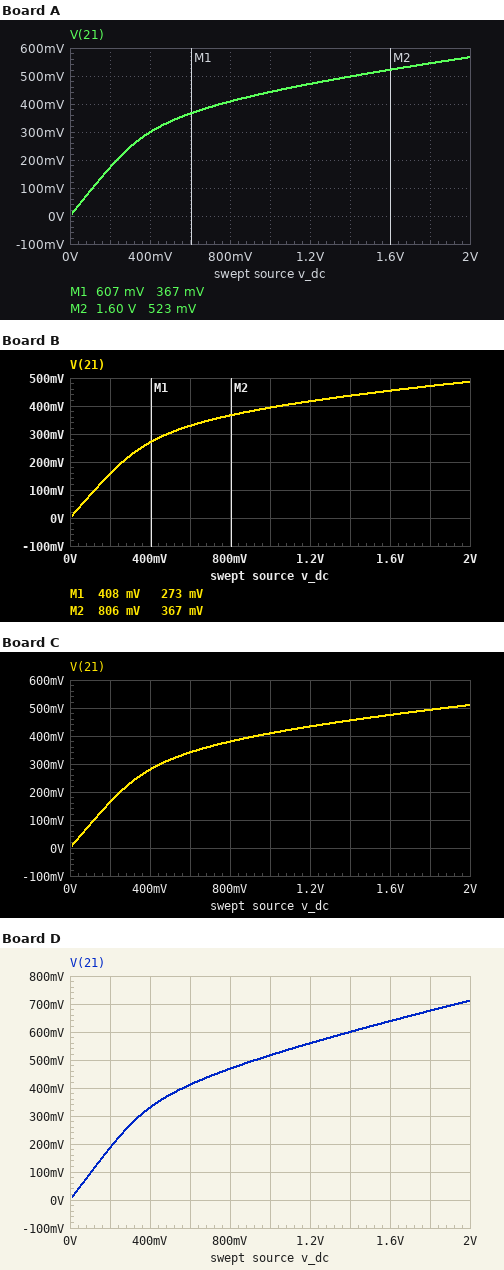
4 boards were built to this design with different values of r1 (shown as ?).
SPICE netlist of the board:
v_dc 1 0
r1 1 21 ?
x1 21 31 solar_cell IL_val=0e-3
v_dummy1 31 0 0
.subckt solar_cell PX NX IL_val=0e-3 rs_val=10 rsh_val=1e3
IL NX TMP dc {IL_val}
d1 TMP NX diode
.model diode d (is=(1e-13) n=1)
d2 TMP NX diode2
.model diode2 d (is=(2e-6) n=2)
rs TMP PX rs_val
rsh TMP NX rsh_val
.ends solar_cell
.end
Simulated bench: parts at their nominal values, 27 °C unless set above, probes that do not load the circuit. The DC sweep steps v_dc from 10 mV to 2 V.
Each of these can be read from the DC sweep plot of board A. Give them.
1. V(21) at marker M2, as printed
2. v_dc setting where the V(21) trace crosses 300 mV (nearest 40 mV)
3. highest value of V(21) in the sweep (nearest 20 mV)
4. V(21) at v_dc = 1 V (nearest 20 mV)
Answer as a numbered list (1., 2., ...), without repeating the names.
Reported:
1. 523 mV
2. 400 mV
3. 560 mV
4. 440 mV
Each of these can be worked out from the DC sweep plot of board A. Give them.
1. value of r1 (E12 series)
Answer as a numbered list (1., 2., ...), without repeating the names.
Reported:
1. 120 Ω
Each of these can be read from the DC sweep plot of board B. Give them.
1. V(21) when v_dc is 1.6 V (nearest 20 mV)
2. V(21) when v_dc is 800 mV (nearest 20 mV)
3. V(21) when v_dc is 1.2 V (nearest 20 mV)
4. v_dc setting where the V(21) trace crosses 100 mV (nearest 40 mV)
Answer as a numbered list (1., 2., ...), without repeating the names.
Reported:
1. 460 mV
2. 360 mV
3. 420 mV
4. 120 mV
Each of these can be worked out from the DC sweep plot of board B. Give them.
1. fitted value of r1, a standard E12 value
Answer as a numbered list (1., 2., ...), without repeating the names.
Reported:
1. 220 Ω
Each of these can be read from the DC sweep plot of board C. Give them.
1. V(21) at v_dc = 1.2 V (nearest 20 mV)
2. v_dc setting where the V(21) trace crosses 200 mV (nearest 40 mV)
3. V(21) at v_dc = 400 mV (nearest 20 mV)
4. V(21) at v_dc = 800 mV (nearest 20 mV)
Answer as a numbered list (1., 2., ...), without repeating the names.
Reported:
1. 440 mV
2. 240 mV
3. 280 mV
4. 380 mV
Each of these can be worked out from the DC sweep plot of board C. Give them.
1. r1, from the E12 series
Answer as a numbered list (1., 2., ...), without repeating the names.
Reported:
1. 180 Ω
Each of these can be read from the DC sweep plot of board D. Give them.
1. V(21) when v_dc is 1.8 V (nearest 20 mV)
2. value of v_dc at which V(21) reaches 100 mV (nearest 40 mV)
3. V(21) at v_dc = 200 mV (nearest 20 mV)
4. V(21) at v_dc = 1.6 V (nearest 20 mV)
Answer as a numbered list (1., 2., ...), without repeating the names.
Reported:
1. 680 mV
2. 120 mV
3. 180 mV
4. 640 mV
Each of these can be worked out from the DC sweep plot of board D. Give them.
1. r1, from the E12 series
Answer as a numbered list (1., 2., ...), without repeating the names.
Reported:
1. 56 Ω
